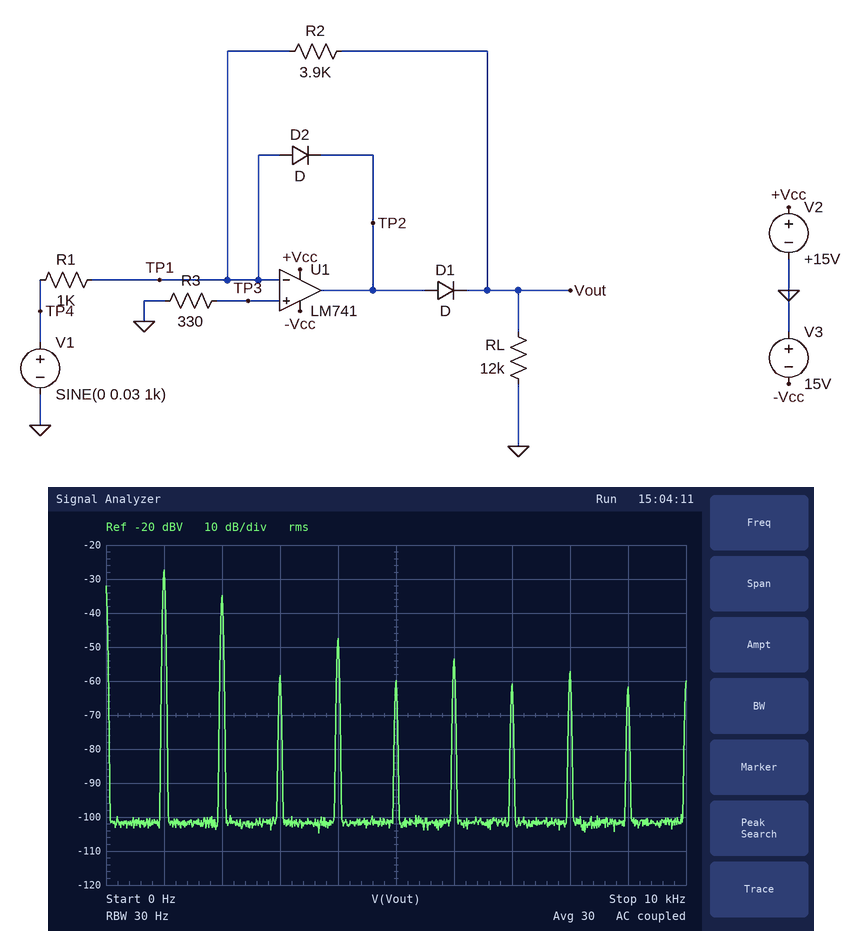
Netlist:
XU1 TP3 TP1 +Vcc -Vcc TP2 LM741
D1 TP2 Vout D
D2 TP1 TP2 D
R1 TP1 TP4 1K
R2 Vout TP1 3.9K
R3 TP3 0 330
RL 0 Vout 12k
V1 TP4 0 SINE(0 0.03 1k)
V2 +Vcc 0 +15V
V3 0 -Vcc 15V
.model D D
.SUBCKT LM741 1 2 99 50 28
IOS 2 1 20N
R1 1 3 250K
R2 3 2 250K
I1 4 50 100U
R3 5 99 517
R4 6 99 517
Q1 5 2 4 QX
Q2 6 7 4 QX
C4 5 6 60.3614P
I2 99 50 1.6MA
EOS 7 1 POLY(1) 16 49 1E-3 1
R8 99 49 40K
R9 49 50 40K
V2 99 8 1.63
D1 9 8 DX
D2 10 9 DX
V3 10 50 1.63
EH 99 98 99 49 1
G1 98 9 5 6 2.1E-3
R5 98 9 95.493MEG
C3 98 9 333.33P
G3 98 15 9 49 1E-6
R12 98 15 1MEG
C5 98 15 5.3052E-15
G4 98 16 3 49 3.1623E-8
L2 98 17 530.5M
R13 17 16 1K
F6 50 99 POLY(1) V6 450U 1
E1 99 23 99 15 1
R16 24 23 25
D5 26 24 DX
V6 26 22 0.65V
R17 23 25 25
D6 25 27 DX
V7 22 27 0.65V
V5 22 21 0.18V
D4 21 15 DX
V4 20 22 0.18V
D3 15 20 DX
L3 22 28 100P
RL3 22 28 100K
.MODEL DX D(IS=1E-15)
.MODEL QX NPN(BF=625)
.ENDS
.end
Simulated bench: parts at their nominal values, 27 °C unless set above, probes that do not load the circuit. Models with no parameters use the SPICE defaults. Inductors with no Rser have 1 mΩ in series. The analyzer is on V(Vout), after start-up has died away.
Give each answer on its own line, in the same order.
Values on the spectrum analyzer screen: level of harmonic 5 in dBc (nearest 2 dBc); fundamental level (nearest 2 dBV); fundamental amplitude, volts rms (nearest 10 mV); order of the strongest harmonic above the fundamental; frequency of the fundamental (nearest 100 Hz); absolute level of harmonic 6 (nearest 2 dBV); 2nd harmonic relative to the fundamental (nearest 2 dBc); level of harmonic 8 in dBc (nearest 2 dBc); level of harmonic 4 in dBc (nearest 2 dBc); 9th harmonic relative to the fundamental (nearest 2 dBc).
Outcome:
-32 dBc
-28 dBV
40 mV
2
1.0 kHz
-54 dBV
-8 dBc
-30 dBc
-20 dBc
-34 dBc
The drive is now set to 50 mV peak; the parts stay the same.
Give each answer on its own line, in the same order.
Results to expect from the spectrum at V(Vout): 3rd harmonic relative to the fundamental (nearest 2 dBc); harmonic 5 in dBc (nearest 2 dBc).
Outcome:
-34 dBc
-36 dBc
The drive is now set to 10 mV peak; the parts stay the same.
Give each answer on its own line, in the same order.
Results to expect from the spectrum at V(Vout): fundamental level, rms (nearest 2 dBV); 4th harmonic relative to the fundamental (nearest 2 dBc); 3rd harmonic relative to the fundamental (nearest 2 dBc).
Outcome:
-36 dBV
-18 dBc
-24 dBc
